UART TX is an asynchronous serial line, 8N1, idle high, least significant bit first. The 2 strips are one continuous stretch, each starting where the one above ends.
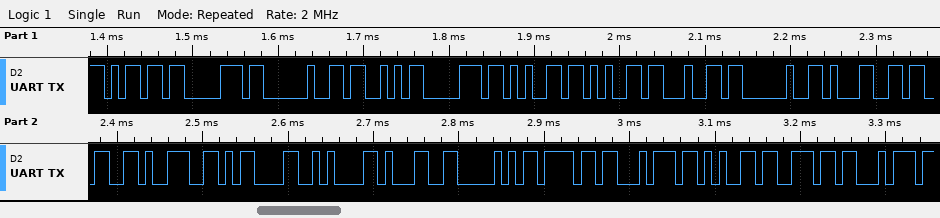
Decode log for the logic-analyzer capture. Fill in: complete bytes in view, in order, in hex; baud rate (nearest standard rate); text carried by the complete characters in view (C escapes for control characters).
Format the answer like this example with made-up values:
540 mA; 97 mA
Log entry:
6D 70 20 53 70 65 65 64 20 31 33 39 0D 0A 31 50 6F 74 65 6E 74; 115200 baud; "mp Speed 139\r\n1Potent"
